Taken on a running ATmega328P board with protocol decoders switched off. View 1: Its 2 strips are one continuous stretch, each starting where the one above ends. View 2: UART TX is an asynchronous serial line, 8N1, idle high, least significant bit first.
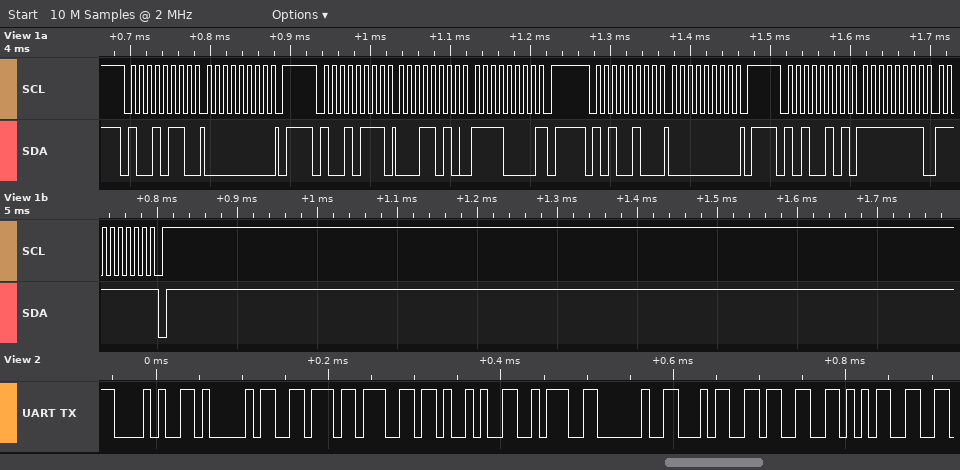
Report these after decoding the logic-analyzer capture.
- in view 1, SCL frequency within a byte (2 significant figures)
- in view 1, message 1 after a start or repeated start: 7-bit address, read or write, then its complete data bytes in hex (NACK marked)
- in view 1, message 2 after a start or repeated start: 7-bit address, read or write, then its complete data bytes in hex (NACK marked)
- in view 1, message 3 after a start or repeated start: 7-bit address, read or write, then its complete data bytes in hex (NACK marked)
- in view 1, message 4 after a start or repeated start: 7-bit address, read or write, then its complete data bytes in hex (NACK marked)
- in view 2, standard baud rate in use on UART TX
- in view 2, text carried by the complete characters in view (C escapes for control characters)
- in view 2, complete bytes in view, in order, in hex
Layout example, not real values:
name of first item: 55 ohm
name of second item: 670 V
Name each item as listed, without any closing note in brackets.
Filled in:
in view 1, SCL frequency within a byte: 100 kHz
in view 1, message 1 after a start or repeated start: 7-bit address, read or write, then its complete data bytes in hex: 0x4B write: 00
in view 1, message 2 after a start or repeated start: 7-bit address, read or write, then its complete data bytes in hex: 0x4B read: 1A F0 NACK
in view 1, message 3 after a start or repeated start: 7-bit address, read or write, then its complete data bytes in hex: 0x52 write: 00
in view 1, message 4 after a start or repeated start: 7-bit address, read or write, then its complete data bytes in hex: 0x52 read: FF FF NACK
in view 2, standard baud rate in use on UART TX: 115200 baud
in view 2, text carried by the complete characters in view: "(Avg): 435"
in view 2, complete bytes in view, in order, in hex: 0x28 0x41 0x76 0x67 0x29 0x3A 0x20 0x34 0x33 0x35
